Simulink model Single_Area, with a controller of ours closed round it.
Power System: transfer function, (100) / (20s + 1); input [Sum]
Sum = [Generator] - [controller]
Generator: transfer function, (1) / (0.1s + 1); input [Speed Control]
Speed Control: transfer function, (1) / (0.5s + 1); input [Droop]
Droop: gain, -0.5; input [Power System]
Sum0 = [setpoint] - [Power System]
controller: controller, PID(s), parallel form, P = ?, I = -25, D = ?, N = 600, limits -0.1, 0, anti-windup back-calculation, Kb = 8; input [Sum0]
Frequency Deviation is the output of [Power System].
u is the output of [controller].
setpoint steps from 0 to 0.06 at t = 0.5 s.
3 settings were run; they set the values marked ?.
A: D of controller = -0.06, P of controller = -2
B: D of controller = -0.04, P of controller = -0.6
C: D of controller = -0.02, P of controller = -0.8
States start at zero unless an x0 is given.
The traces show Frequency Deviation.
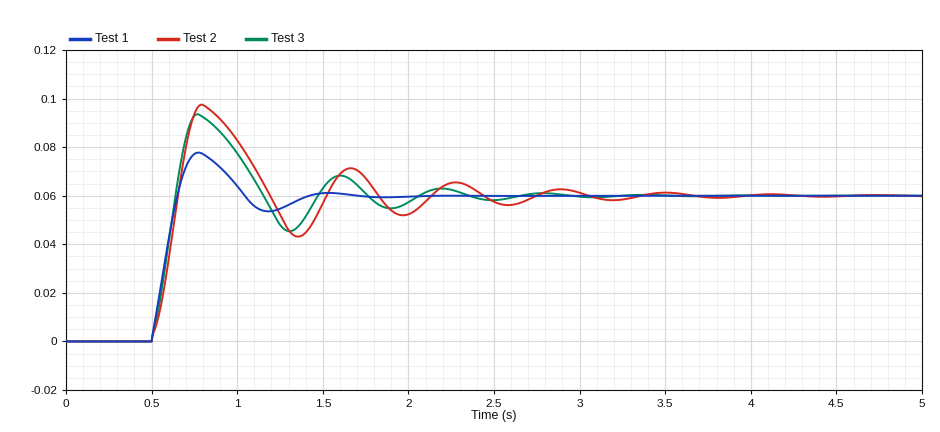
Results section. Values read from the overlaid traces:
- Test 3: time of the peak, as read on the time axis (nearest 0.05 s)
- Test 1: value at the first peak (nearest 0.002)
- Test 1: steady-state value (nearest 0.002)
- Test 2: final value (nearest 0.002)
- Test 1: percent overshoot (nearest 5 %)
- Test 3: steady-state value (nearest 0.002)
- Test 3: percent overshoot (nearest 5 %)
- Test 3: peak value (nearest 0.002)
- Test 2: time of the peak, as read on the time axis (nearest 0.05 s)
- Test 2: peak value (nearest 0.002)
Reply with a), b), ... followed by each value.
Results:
a) 0.75 s
b) 0.078
c) 0.060
d) 0.060
e) 30 %
f) 0.060
g) 55 %
h) 0.094
i) 0.80 s
j) 0.098
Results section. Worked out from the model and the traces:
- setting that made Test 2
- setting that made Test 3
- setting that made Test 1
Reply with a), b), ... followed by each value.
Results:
a) B
b) C
c) A
